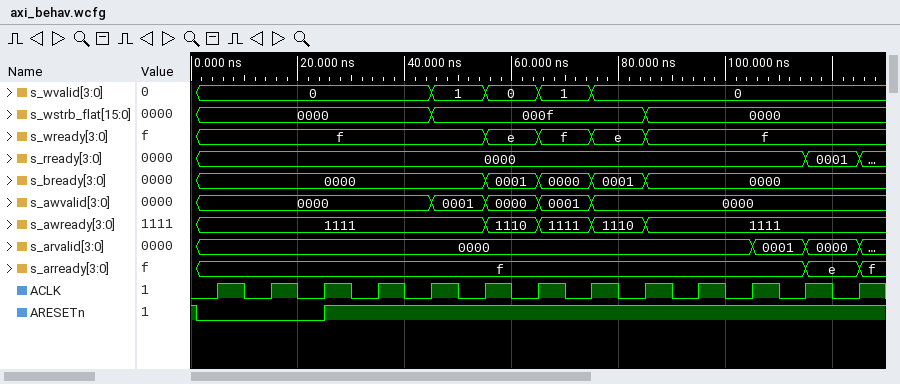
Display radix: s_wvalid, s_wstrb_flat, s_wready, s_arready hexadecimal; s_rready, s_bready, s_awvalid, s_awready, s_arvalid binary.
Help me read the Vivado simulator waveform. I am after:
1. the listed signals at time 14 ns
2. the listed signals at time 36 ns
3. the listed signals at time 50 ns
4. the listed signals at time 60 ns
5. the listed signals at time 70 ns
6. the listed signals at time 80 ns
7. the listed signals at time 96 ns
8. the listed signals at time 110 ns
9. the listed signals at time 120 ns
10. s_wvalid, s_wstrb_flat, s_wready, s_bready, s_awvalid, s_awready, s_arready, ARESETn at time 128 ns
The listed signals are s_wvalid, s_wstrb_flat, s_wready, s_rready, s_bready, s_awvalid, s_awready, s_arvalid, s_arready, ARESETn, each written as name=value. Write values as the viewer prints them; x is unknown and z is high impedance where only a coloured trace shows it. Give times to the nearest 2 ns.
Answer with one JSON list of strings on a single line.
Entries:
["s_wvalid=0, s_wstrb_flat=0000, s_wready=f, s_rready=0000, s_bready=0000, s_awvalid=0000, s_awready=1111, s_arvalid=0000, s_arready=f, ARESETn=0", "s_wvalid=0, s_wstrb_flat=0000, s_wready=f, s_rready=0000, s_bready=0000, s_awvalid=0000, s_awready=1111, s_arvalid=0000, s_arready=f, ARESETn=1", "s_wvalid=1, s_wstrb_flat=000f, s_wready=f, s_rready=0000, s_bready=0000, s_awvalid=0001, s_awready=1111, s_arvalid=0000, s_arready=f, ARESETn=1", "s_wvalid=0, s_wstrb_flat=000f, s_wready=e, s_rready=0000, s_bready=0001, s_awvalid=0000, s_awready=1110, s_arvalid=0000, s_arready=f, ARESETn=1", "s_wvalid=1, s_wstrb_flat=000f, s_wready=f, s_rready=0000, s_bready=0000, s_awvalid=0001, s_awready=1111, s_arvalid=0000, s_arready=f, ARESETn=1", "s_wvalid=0, s_wstrb_flat=000f, s_wready=e, s_rready=0000, s_bready=0001, s_awvalid=0000, s_awready=1110, s_arvalid=0000, s_arready=f, ARESETn=1", "s_wvalid=0, s_wstrb_flat=0000, s_wready=f, s_rready=0000, s_bready=0000, s_awvalid=0000, s_awready=1111, s_arvalid=0000, s_arready=f, ARESETn=1", "s_wvalid=0, s_wstrb_flat=0000, s_wready=f, s_rready=0000, s_bready=0000, s_awvalid=0000, s_awready=1111, s_arvalid=0001, s_arready=f, ARESETn=1", "s_wvalid=0, s_wstrb_flat=0000, s_wready=f, s_rready=0001, s_bready=0000, s_awvalid=0000, s_awready=1111, s_arvalid=0000, s_arready=e, ARESETn=1", "s_wvalid=0, s_wstrb_flat=0000, s_wready=f, s_bready=0000, s_awvalid=0000, s_awready=1111, s_arready=f, ARESETn=1"]
